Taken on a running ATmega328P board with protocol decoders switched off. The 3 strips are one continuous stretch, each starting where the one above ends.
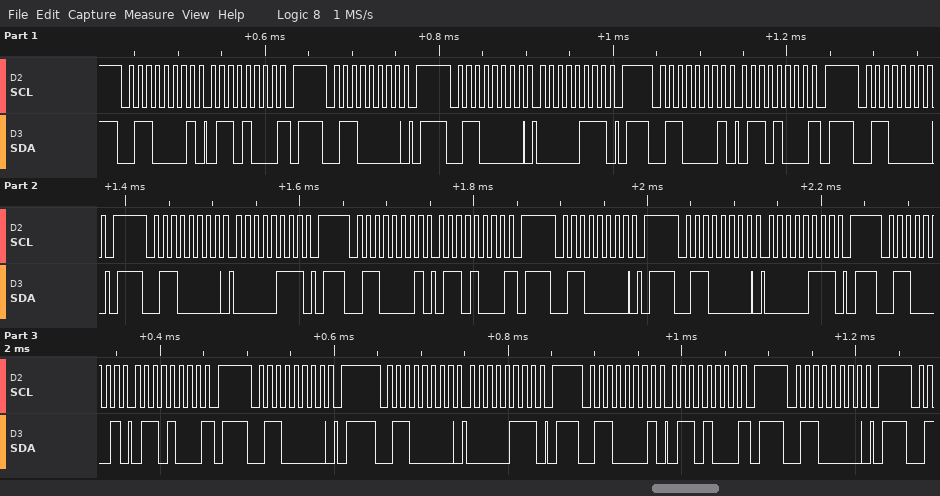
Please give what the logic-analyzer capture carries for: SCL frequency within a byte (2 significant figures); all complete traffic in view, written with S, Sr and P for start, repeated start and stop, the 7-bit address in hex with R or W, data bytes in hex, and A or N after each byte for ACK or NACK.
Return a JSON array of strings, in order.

["100 kHz", "S 30R A 68 N P S 30W A P S 30W A 07 A P S 30R A 68 N P S 30W A P S 30W A 07 A P S 30R A 68 N P S 30W A P S 30W A 07 A P S 30R A 68 N P S 30W A P S 30W A 07 A P S 30R A 68 N P S 30W A P"]
